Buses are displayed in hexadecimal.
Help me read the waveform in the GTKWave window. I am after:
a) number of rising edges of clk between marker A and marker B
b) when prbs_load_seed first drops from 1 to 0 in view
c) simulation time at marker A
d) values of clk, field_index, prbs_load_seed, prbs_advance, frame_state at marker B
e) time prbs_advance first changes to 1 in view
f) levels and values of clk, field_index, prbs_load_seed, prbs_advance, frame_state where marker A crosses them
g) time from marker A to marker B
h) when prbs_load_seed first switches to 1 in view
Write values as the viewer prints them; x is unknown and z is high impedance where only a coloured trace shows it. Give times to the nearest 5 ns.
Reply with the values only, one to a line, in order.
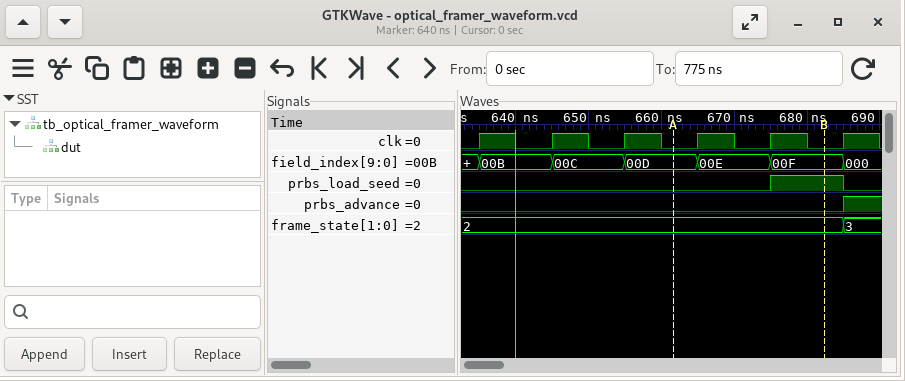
2
685 ns
660 ns
clk=0, field_index=00F, prbs_load_seed=1, prbs_advance=0, frame_state=2
685 ns
clk=0, field_index=00D, prbs_load_seed=0, prbs_advance=0, frame_state=2
20 ns
675 ns
